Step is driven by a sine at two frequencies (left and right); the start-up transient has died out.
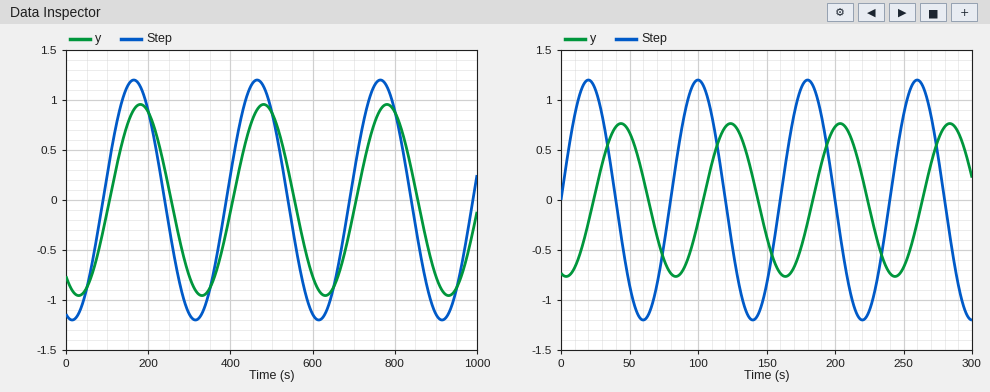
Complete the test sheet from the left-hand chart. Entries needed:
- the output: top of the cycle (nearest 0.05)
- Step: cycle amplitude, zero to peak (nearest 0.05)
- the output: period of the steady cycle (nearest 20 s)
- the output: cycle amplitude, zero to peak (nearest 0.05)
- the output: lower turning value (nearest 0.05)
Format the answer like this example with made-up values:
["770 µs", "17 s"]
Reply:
["0.95", "1.20", "300 s", "0.95", "-0.95"]
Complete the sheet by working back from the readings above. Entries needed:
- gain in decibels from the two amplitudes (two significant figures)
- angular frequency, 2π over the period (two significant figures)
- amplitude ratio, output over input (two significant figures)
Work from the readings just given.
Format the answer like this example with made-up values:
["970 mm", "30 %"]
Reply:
["-2.0 dB", "0.021 rad/s", "0.79"]
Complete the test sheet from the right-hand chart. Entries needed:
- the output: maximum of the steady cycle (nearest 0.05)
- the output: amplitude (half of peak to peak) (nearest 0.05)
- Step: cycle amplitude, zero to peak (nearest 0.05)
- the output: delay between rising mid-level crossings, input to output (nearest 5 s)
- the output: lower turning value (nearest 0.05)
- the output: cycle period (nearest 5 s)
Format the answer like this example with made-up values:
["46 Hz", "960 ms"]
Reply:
["0.75", "0.75", "1.20", "25 s", "-0.75", "80 s"]
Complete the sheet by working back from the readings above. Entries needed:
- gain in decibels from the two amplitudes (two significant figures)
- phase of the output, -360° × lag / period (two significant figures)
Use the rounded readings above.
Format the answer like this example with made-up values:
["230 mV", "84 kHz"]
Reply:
["-4.1 dB", "-110°"]
